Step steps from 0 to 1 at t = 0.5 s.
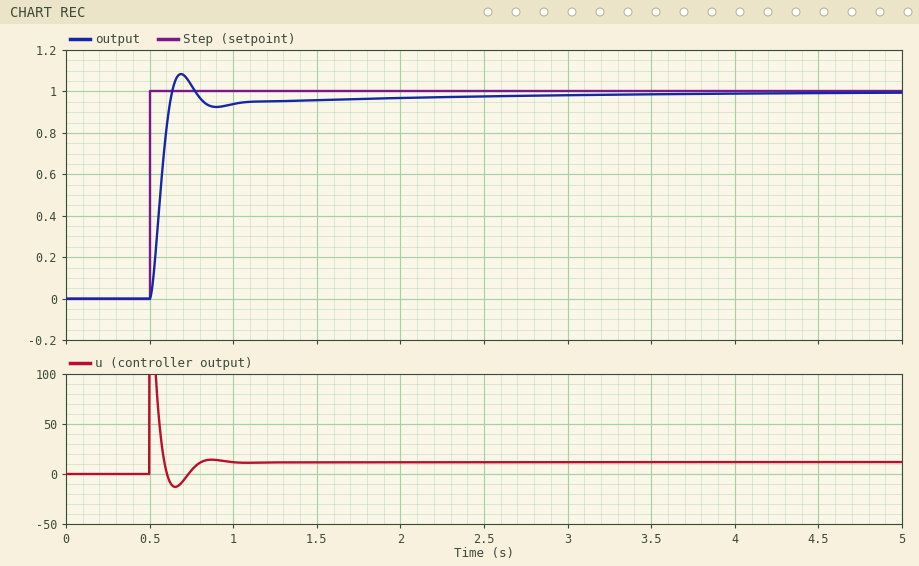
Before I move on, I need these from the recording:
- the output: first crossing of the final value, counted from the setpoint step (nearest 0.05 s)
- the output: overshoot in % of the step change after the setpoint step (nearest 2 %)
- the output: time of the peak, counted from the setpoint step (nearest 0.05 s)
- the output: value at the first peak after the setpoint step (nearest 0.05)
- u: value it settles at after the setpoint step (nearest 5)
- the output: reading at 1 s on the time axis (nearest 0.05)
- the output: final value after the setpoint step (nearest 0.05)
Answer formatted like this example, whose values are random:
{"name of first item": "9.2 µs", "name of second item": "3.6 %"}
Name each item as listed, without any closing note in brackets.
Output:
{"the output: first crossing of the final value, counted from the setpoint step": "0.15 s", "the output: overshoot in % of the step change after the setpoint step": "8 %", "the output: time of the peak, counted from the setpoint step": "0.20 s", "the output: value at the first peak after the setpoint step": "1.10", "u: value it settles at after the setpoint step": "10", "the output: reading at 1 s on the time axis": "0.95", "the output: final value after the setpoint step": "1.00"}
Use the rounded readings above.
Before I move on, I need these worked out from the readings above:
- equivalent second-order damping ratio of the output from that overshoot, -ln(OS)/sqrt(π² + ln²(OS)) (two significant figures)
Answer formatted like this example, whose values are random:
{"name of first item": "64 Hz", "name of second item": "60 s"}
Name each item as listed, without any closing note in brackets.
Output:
{"equivalent second-order damping ratio of the output from that overshoot, -ln(OS)/sqrt(π² + ln²(OS))": "0.63"}
